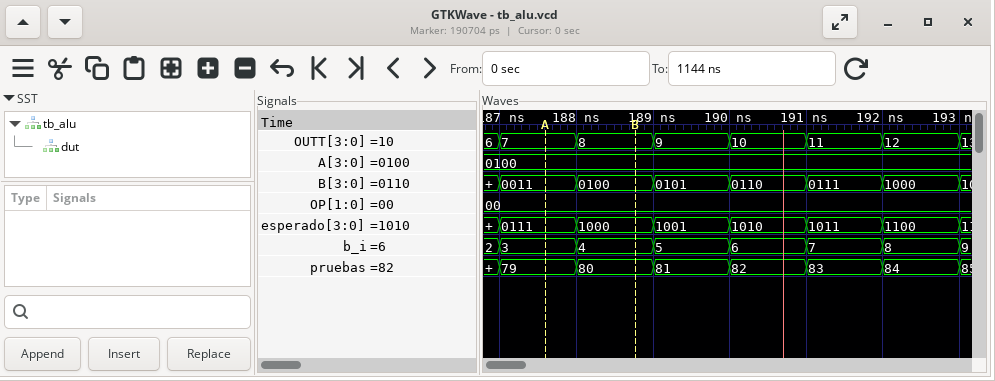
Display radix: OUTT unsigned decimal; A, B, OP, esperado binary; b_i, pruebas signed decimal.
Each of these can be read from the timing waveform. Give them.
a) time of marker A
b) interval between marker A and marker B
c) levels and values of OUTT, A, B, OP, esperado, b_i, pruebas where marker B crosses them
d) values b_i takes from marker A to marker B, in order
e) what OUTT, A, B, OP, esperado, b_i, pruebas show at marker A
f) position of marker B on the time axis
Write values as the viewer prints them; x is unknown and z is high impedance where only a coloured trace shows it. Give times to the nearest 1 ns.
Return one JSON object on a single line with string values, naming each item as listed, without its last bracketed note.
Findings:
{"time of marker A": "188 ns", "interval between marker A and marker B": "1 ns", "levels and values of OUTT, A, B, OP, esperado, b_i, pruebas where marker B crosses them": "OUTT=8, A=0100, B=0100, OP=00, esperado=1000, b_i=4, pruebas=80", "values b_i takes from marker A to marker B, in order": "3, 4", "what OUTT, A, B, OP, esperado, b_i, pruebas show at marker A": "OUTT=7, A=0100, B=0011, OP=00, esperado=0111, b_i=3, pruebas=79", "position of marker B on the time axis": "189 ns"}
